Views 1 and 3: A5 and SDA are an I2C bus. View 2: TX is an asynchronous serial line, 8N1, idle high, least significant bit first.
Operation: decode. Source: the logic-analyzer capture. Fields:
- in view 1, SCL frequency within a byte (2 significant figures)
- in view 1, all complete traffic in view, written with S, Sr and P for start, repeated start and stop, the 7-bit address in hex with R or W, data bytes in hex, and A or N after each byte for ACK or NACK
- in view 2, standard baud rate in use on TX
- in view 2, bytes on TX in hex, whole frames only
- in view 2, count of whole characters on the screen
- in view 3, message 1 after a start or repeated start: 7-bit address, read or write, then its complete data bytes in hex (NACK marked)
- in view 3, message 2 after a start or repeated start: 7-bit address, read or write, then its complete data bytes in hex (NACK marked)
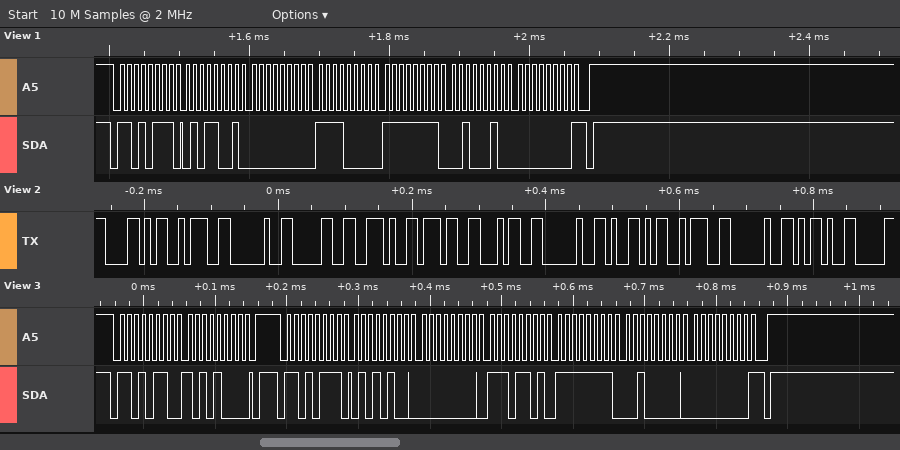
100 kHz
S 6BR A 59 A 00 A F0 A FF A 22 A 00 N P
115200 baud
58 3A 20 30 2E 37 34 20 59 3A 20 2D
12
0x6B write: A8
0x6B read: 54 00 ED FF 20 00 NACK
